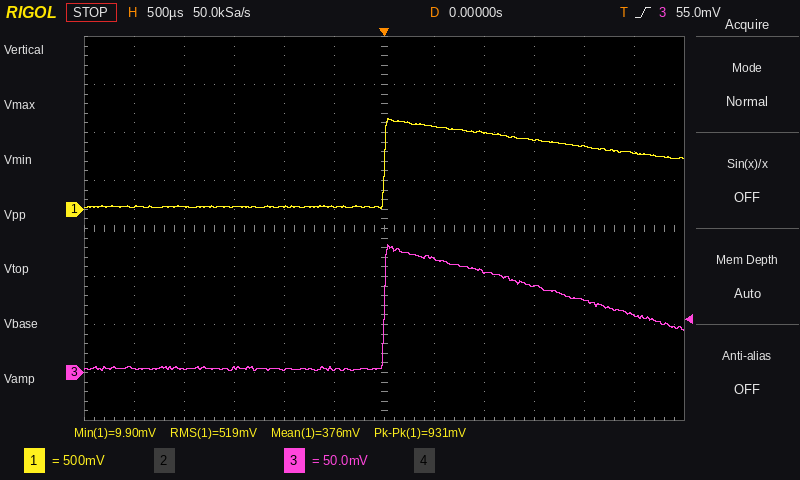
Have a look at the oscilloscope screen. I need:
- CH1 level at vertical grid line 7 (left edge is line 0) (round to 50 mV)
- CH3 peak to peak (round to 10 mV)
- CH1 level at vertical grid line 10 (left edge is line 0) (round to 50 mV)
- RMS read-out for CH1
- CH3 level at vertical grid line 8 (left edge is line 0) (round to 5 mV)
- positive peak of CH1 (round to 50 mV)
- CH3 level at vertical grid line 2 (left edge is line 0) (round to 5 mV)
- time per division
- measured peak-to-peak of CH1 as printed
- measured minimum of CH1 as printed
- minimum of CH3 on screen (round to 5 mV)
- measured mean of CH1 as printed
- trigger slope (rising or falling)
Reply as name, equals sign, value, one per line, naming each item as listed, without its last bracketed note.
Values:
CH1 level at vertical grid line 7 (left edge is line 0) = 850 mV
CH3 peak to peak = 130 mV
CH1 level at vertical grid line 10 (left edge is line 0) = 650 mV
RMS read-out for CH1 = 519 mV
CH3 level at vertical grid line 8 (left edge is line 0) = 105 mV
positive peak of CH1 = 950 mV
CH3 level at vertical grid line 2 (left edge is line 0) = 5 mV
time per division = 500 µs
measured peak-to-peak of CH1 as printed = 931 mV
measured minimum of CH1 as printed = 9.90 mV
minimum of CH3 on screen = 0 mV
measured mean of CH1 as printed = 376 mV
trigger slope = rising
